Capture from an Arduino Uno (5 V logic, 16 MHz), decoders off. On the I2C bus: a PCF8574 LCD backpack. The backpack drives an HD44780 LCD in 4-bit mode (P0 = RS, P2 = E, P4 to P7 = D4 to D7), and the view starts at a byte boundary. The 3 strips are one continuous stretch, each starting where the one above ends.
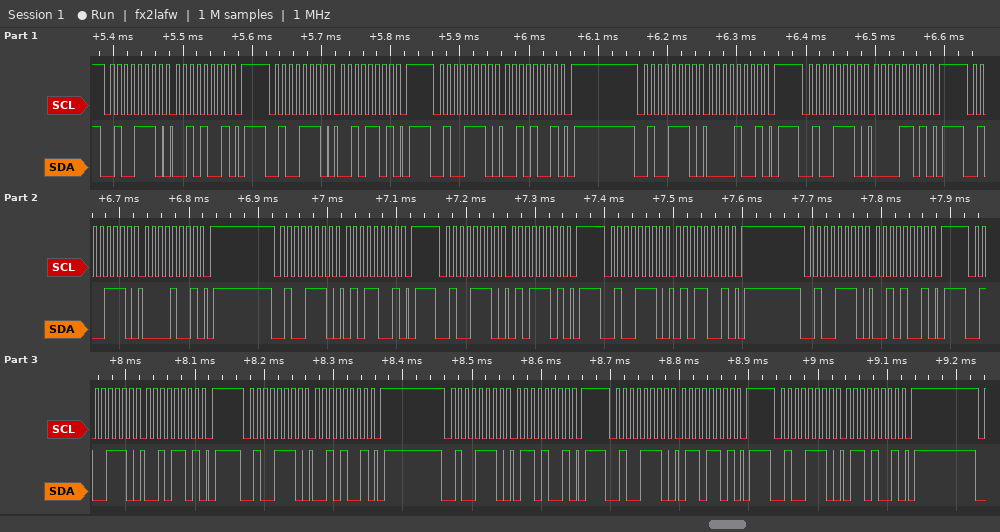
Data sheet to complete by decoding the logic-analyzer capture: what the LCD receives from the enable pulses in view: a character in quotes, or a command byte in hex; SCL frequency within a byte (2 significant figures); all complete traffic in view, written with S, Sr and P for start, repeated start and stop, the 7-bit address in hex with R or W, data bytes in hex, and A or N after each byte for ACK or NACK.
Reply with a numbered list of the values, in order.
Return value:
1. ' ' 'R'
2. 100 kHz
3. S 27W A 29 A P S 27W A 2D A P S 27W A 29 A P S 27W A 09 A P S 27W A 0D A P S 27W A 09 A P S 27W A 59 A P S 27W A 5D A P S 27W A 59 A P S 27W A 29 A P S 27W A 2D A P S 27W A 29 A P S 27W A 69 A P S 27W A 6D A P S 27W A 69 A P
